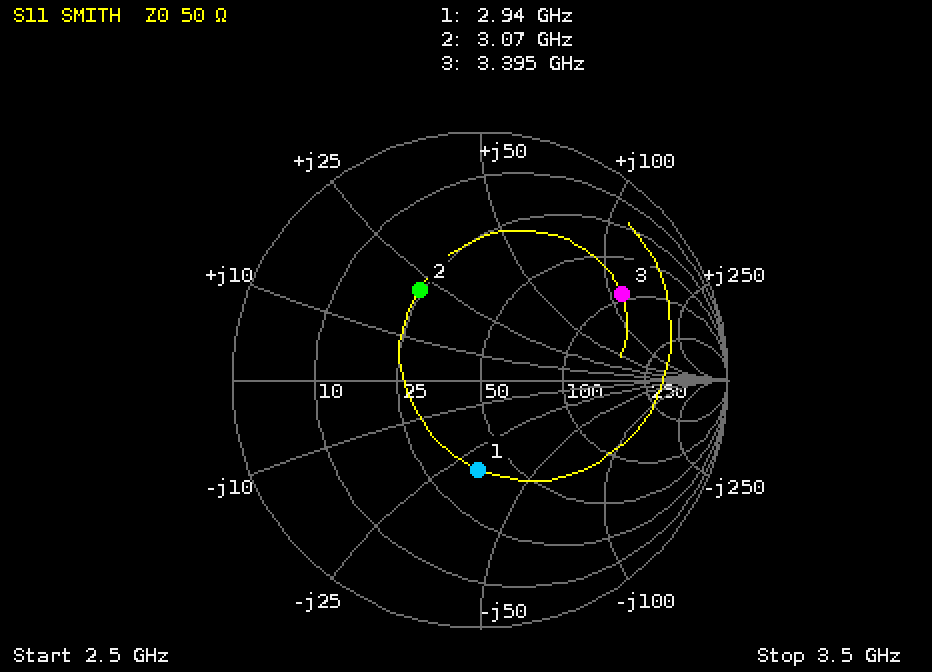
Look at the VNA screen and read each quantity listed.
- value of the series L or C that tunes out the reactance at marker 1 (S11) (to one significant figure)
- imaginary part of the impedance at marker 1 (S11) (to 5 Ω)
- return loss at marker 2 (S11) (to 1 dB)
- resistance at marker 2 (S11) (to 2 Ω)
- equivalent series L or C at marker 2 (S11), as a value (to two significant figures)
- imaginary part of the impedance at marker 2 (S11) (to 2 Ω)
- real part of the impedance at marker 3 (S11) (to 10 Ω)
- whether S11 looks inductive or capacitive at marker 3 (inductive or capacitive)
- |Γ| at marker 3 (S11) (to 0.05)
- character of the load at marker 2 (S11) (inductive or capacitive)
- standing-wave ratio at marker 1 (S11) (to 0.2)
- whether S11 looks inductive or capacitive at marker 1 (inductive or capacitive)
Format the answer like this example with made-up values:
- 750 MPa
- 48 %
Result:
- 2 nH
- -30 Ω
- 7 dB
- 24 Ω
- 1.1 nH
- +22 Ω
- 90 Ω
- inductive
- 0.65
- inductive
- 2.2
- capacitive
